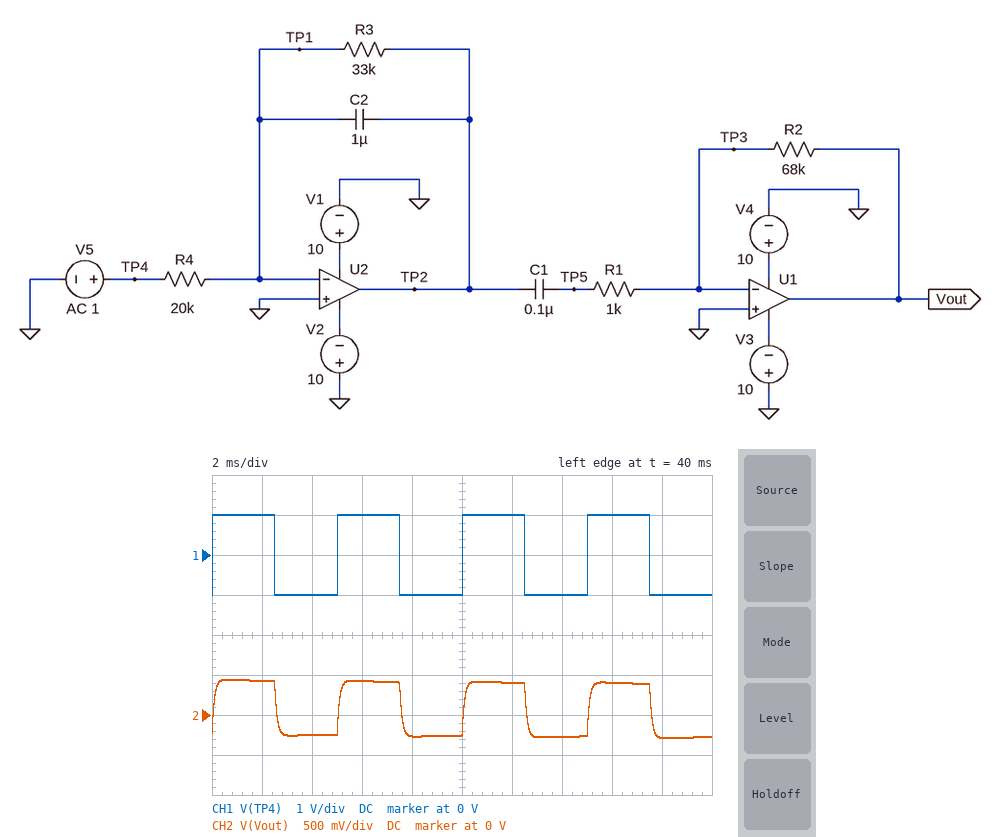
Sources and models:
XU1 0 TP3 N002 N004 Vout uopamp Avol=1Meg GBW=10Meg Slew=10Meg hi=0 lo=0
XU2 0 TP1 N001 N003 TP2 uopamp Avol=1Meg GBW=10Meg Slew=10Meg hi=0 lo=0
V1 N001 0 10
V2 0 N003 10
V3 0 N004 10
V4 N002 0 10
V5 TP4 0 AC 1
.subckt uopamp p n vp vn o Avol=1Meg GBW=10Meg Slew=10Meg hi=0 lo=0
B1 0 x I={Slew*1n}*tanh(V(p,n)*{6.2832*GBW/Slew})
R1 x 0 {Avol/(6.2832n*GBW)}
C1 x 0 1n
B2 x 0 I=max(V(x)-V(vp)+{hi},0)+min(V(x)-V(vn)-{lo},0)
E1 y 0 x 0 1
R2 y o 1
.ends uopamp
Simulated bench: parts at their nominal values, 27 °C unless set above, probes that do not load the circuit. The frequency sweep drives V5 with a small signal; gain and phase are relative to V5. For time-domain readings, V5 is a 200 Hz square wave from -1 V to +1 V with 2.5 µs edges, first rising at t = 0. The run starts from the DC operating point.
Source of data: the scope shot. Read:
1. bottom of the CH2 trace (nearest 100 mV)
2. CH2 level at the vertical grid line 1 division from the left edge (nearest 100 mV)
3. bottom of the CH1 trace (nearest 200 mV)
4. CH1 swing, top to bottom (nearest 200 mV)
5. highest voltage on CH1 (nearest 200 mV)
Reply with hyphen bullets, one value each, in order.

- -300 mV
- 400 mV
- -1.0 V
- 2.0 V
- 1.0 V
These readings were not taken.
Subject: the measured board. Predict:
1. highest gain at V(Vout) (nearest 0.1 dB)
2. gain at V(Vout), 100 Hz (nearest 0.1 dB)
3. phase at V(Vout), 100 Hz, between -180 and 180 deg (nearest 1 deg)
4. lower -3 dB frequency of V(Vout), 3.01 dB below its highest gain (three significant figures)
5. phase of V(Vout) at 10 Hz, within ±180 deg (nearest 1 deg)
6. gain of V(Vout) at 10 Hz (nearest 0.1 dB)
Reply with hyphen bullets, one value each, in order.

- -9.4 dB
- -9.4 dB
- -1 deg
- 4.79 Hz
- 25 deg
- -10.3 dB
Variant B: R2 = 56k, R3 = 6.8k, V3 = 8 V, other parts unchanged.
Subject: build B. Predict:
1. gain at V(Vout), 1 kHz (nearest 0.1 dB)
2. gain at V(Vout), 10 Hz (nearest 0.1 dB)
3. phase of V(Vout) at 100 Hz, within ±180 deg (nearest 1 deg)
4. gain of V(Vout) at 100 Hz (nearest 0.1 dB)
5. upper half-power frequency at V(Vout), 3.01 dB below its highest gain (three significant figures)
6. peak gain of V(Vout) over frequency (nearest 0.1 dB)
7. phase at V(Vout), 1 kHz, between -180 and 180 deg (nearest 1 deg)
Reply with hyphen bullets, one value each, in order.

- -12.5 dB
- -19.2 dB
- 10 deg
- -11.3 dB
- 1.65 kHz
- -11.2 dB
- -31 deg
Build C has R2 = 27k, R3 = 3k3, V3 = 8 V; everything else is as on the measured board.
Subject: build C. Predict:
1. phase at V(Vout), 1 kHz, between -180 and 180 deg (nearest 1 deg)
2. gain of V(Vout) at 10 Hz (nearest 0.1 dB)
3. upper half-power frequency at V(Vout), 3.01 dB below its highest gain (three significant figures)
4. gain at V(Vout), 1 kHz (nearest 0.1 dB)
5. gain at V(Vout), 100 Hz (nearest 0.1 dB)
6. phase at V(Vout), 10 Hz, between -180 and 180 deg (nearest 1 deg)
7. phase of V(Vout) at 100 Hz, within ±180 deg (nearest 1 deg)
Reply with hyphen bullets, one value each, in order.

- -29 deg
- -31.2 dB
- 1.69 kHz
- -18.8 dB
- -18.3 dB
- 78 deg
- 22 deg
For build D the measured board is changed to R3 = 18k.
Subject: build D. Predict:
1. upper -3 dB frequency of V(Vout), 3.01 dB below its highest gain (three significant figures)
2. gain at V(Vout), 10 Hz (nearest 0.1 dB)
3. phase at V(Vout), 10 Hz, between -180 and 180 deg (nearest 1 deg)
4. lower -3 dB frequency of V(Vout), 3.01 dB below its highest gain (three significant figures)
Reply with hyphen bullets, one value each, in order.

- 1.63 kHz
- -11.9 dB
- 41 deg
- 8.75 Hz
